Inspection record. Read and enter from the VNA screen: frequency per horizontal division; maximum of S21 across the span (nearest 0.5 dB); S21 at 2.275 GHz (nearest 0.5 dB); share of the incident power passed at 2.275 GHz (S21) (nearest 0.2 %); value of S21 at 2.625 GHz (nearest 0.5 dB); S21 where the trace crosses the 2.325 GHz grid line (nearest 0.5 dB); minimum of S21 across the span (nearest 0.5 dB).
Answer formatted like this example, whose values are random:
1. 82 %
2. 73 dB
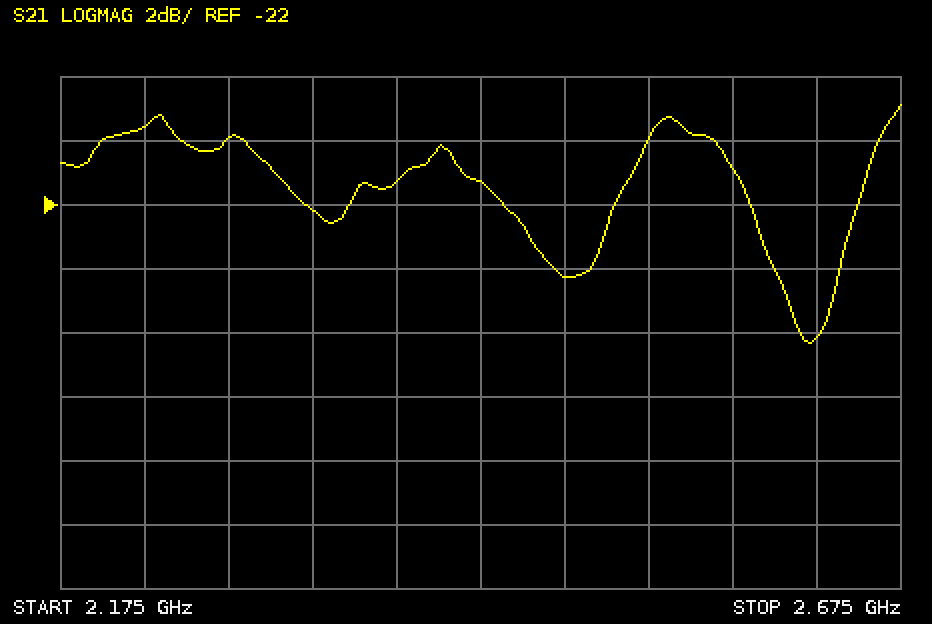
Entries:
1. 50 MHz
2. -19.0 dB
3. -20.0 dB
4. 1.0 %
5. -26.0 dB
6. -22.0 dB
7. -26.5 dB
